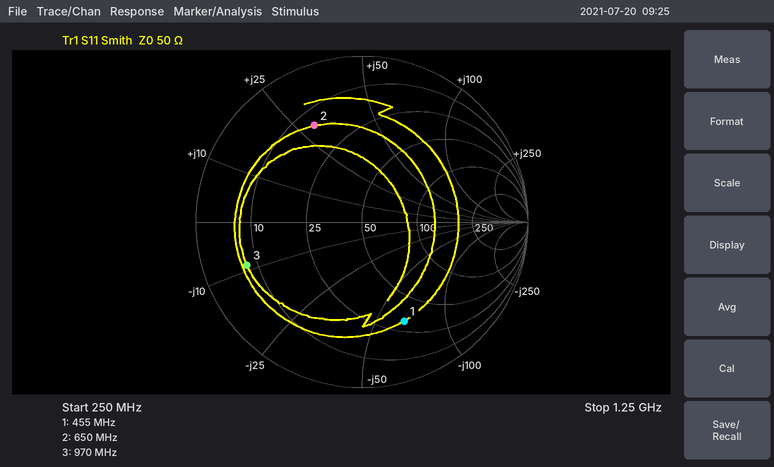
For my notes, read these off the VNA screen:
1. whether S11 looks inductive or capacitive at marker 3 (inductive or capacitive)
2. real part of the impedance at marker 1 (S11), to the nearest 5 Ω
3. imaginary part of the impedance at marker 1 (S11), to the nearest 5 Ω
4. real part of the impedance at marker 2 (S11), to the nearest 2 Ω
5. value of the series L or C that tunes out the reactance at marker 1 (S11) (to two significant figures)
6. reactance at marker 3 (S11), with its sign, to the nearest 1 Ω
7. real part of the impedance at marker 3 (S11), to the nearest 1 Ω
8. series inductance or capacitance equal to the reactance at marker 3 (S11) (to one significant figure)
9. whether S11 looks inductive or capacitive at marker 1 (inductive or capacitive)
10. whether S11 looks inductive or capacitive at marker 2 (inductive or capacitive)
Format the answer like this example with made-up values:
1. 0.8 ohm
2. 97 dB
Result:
1. capacitive
2. 30 Ω
3. -65 Ω
4. 14 Ω
5. 23 nH
6. -9 Ω
7. 8 Ω
8. 20 pF
9. capacitive
10. inductive
